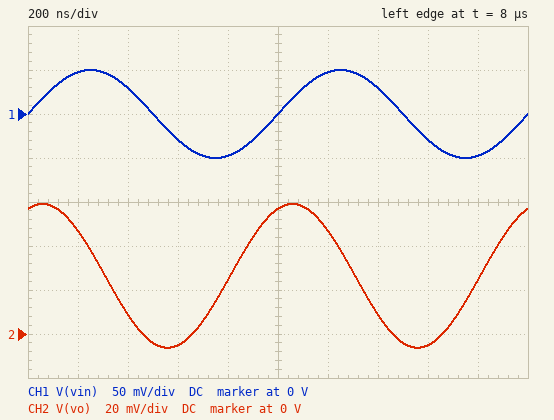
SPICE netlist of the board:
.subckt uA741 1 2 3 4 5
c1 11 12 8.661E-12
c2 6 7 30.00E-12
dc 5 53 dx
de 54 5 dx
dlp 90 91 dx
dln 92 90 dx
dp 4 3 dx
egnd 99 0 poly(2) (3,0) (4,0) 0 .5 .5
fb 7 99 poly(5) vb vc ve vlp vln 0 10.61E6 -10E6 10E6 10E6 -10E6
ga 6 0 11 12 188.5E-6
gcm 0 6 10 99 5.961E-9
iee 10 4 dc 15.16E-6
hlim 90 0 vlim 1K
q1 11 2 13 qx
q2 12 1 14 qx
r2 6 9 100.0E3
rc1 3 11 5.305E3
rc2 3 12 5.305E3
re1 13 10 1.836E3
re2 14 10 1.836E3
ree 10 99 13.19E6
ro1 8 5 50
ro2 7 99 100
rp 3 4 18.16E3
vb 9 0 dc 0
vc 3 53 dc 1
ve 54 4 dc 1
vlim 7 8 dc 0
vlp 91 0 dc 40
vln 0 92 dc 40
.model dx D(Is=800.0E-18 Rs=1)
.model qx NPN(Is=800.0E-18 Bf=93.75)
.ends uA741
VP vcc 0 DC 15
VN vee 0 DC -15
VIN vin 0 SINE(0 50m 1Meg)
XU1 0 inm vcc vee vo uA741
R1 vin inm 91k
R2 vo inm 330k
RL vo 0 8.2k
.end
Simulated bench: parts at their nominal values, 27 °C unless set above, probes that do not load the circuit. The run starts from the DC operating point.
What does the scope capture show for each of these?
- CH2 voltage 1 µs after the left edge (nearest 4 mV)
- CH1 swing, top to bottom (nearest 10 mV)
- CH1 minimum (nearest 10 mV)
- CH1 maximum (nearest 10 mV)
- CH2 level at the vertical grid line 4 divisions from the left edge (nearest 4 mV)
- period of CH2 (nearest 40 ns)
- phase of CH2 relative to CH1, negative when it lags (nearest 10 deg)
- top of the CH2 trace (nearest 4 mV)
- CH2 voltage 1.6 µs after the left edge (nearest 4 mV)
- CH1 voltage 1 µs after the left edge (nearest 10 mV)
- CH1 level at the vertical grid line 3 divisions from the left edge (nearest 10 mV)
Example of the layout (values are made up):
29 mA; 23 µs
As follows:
56 mV; 100 mV; -50 mV; 50 mV; 24 mV; 1.00 µs; 70 deg; 60 mV; -4 mV; 0 V; -30 mV
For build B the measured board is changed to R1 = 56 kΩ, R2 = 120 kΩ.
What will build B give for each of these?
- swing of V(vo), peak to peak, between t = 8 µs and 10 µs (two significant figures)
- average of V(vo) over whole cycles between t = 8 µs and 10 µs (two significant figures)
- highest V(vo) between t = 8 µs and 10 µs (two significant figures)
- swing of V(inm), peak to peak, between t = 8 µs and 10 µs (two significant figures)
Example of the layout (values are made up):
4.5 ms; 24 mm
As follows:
61 mV; 9.6 mV; 40 mV; 73 mV
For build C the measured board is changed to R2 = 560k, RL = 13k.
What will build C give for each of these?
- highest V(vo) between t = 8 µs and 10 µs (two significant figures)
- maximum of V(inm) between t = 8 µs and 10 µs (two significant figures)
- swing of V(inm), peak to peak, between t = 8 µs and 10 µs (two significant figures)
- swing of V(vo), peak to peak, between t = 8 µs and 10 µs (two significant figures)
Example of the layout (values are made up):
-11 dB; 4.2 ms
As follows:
79 mV; 42 mV; 84 mV; 69 mV
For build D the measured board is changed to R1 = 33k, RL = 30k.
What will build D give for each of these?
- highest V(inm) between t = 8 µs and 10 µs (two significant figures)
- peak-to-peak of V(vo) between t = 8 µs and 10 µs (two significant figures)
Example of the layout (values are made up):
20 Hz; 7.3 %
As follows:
46 mV; 75 mV
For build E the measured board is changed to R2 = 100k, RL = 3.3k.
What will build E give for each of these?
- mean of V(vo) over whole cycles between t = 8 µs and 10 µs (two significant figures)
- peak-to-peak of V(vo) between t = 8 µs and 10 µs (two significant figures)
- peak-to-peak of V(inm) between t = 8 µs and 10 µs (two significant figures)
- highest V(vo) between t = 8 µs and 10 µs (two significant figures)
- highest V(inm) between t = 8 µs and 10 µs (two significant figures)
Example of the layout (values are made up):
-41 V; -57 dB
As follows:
8.0 mV; 48 mV; 57 mV; 32 mV; 29 mV
